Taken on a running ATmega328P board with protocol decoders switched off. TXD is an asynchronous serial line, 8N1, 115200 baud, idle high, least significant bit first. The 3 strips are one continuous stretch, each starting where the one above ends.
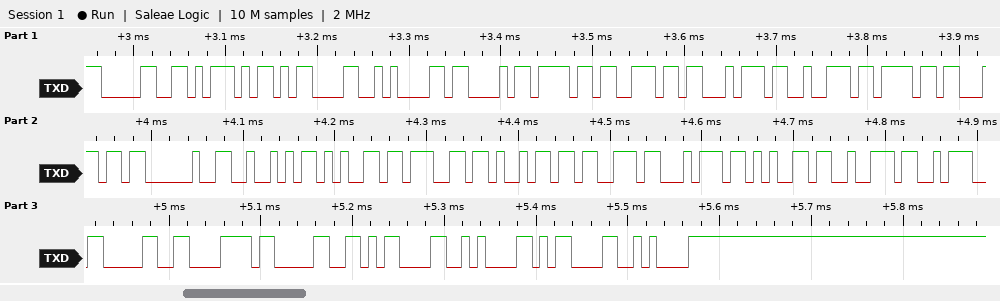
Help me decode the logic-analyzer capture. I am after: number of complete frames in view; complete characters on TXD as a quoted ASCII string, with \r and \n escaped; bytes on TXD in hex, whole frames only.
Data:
28
"0]\r\nControl Register:0x0\r\n\r\n"
30 5D 0D 0A 43 6F 6E 74 72 6F 6C 20 52 65 67 69 73 74 65 72 3A 30 78 30 0D 0A 0D 0A
